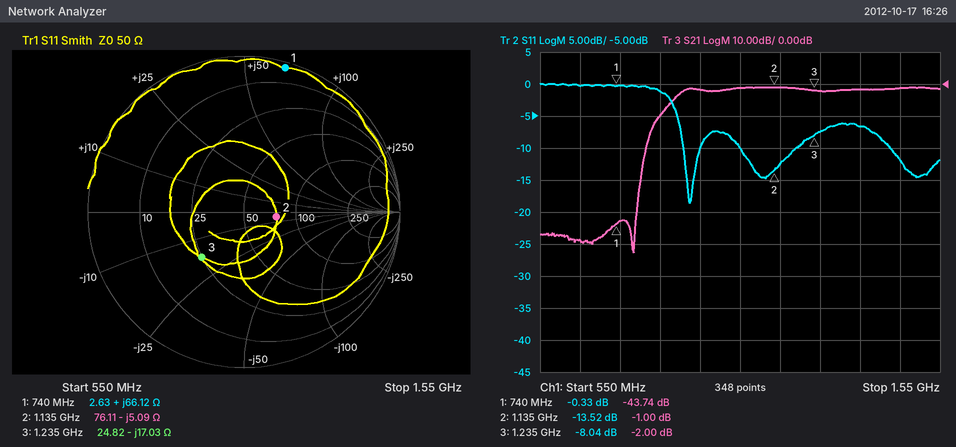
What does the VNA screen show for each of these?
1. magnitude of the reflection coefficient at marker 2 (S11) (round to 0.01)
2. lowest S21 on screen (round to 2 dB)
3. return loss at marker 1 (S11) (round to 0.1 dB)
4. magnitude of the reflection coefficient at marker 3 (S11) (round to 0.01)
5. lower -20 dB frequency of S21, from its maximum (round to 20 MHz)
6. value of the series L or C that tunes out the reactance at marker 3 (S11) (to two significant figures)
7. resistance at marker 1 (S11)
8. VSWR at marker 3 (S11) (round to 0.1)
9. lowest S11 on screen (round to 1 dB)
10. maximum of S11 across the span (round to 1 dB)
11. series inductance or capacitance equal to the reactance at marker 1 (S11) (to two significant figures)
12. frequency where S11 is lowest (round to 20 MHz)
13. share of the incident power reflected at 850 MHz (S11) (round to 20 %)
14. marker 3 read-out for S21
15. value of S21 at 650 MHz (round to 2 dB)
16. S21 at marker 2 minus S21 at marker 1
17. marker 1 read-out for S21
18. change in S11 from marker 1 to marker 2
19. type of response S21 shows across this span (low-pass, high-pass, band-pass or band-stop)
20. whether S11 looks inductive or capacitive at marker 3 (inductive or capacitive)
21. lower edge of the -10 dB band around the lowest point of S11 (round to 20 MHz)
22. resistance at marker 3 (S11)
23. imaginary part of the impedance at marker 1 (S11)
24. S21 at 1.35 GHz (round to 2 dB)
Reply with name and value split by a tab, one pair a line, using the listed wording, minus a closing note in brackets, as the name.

magnitude of the reflection coefficient at marker 2 (S11)	0.21
lowest S21 on screen	-52 dB
return loss at marker 1 (S11)	0.3 dB
magnitude of the reflection coefficient at marker 3 (S11)	0.40
lower -20 dB frequency of S21, from its maximum	820 MHz
value of the series L or C that tunes out the reactance at marker 3 (S11)	2.2 nH
resistance at marker 1	2.63 Ω
VSWR at marker 3 (S11)	2.3
lowest S11 on screen	-19 dB
maximum of S11 across the span	0 dB
series inductance or capacitance equal to the reactance at marker 1 (S11)	14 nH
frequency where S11 is lowest	920 MHz
share of the incident power reflected at 850 MHz (S11)	80 %
marker 3 read-out for S21	-2.00 dB
value of S21 at 650 MHz	-48 dB
S21 at marker 2 minus S21 at marker 1	42.74 dB
marker 1 read-out for S21	-43.74 dB
change in S11 from marker 1 to marker 2	-13.19 dB
type of response S21 shows across this span	high-pass
whether S11 looks inductive or capacitive at marker 3	capacitive
lower edge of the -10 dB band around the lowest point of S11	900 MHz
resistance at marker 3	24.82 Ω
imaginary part of the impedance at marker 1	+66.12 Ω
S21 at 1.35 GHz	-2 dB
